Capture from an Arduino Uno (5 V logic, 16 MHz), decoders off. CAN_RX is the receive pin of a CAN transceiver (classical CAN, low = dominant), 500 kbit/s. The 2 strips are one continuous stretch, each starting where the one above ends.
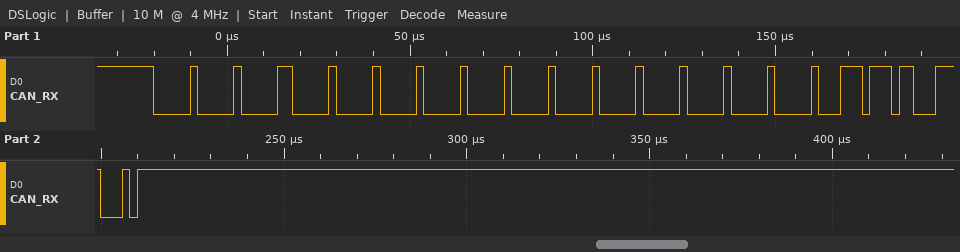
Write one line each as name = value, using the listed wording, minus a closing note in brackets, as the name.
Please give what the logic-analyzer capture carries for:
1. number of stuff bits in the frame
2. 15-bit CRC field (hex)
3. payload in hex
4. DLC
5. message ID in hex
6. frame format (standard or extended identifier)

number of stuff bits in the frame = 15
15-bit CRC field = 0x7638
payload in hex = 00 00 00 00 00 00 00 0E
DLC = 8
message ID in hex = 0x000
frame format = standard
